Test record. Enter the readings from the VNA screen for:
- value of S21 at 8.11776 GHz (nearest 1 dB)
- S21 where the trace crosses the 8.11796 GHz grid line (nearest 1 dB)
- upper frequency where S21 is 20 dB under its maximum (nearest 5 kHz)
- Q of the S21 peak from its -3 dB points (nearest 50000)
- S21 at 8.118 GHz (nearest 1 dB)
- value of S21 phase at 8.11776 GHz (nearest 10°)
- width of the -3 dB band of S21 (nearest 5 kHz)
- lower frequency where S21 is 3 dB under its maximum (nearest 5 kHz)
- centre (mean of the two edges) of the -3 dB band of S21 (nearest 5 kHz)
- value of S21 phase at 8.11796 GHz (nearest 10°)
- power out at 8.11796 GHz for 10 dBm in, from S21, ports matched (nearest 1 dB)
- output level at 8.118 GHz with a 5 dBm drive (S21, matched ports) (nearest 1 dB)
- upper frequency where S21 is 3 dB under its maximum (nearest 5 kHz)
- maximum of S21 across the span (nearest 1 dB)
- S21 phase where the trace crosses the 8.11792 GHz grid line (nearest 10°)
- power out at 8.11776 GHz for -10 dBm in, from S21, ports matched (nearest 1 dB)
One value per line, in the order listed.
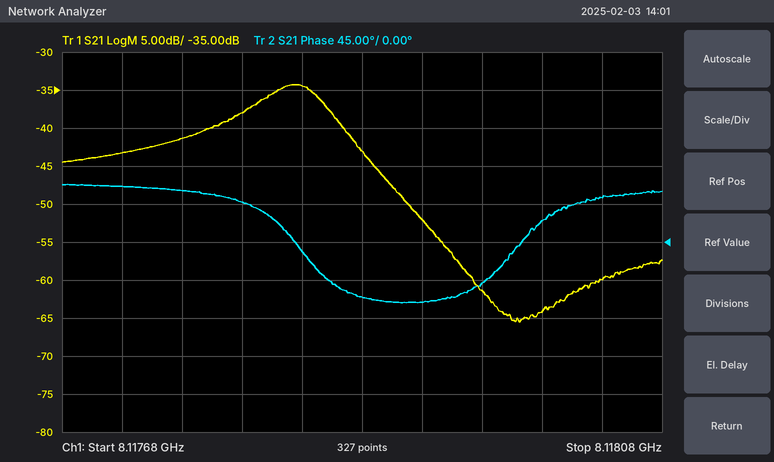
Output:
-41 dB
-61 dB
8.117930 GHz
150000
-64 dB
60°
50 kHz
8.117805 GHz
8.117830 GHz
-50°
-51 dBm
-59 dBm
8.117855 GHz
-34 dB
-70°
-51 dBm
